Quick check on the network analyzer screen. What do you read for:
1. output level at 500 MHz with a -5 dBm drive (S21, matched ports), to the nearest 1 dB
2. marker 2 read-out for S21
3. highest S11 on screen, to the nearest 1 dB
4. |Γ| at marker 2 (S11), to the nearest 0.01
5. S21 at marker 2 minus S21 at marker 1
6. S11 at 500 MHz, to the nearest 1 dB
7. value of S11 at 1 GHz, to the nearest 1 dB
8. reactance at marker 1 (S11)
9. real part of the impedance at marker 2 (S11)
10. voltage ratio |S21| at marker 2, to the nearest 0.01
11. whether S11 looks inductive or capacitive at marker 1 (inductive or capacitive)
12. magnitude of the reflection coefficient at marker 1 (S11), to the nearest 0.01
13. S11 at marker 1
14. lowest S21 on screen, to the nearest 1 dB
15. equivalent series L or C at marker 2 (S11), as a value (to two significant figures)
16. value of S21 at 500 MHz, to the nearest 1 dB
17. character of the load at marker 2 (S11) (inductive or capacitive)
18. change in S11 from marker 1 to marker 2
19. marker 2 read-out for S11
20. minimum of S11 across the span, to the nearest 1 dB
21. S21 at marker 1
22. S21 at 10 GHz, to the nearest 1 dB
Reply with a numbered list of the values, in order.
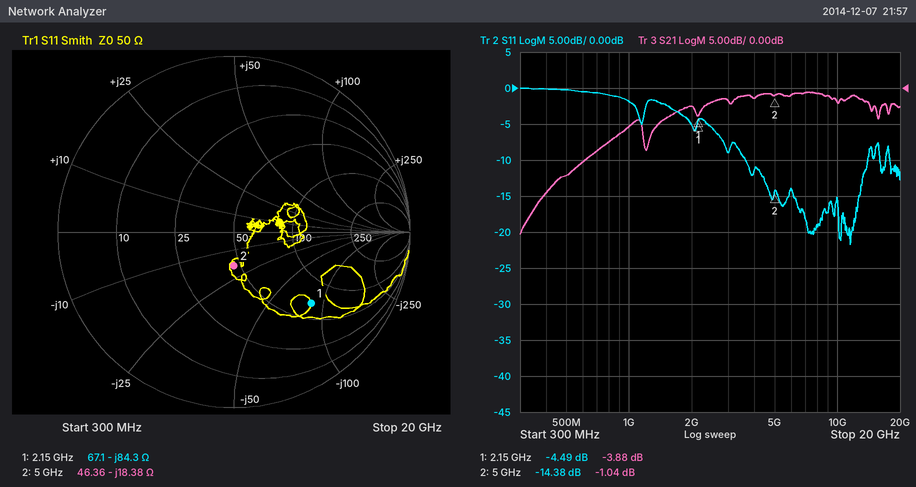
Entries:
1. -17 dBm
2. -1.04 dB
3. 0 dB
4. 0.19
5. 2.84 dB
6. 0 dB
7. -2 dB
8. -84.3 Ω
9. 46.36 Ω
10. 0.89
11. capacitive
12. 0.60
13. -4.49 dB
14. -20 dB
15. 1.7 pF
16. -12 dB
17. capacitive
18. -9.89 dB
19. -14.38 dB
20. -22 dB
21. -3.88 dB
22. -2 dB
